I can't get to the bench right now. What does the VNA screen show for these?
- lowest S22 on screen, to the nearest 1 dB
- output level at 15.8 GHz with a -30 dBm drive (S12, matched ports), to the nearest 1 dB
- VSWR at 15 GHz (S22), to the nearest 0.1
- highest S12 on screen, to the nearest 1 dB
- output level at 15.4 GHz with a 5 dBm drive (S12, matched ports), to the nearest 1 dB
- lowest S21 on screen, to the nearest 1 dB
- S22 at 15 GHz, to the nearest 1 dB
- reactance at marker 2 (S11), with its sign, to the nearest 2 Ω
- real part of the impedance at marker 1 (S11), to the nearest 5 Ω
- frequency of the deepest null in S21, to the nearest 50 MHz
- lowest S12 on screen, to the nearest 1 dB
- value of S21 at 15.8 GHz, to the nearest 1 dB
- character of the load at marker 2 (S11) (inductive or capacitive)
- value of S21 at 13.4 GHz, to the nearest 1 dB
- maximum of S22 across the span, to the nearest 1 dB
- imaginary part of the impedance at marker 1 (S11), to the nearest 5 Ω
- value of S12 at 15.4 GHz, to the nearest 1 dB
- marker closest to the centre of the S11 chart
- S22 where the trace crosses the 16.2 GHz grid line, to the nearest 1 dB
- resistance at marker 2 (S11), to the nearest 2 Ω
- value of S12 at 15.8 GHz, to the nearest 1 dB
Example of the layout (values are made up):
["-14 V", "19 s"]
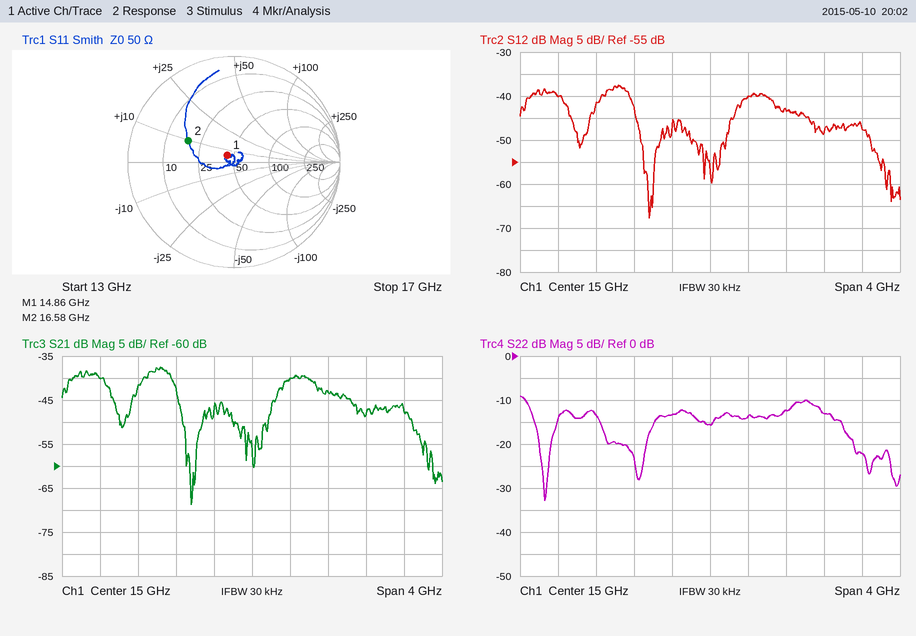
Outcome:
["-33 dB", "-73 dBm", "1.4", "-38 dB", "-35 dBm", "-69 dB", "-16 dB", "+10 Ω", "45 Ω", "14.35 GHz", "-68 dB", "-43 dB", "inductive", "-40 dB", "-9 dB", "+5 Ω", "-40 dB", "marker 1", "-13 dB", "18 Ω", "-43 dB"]
